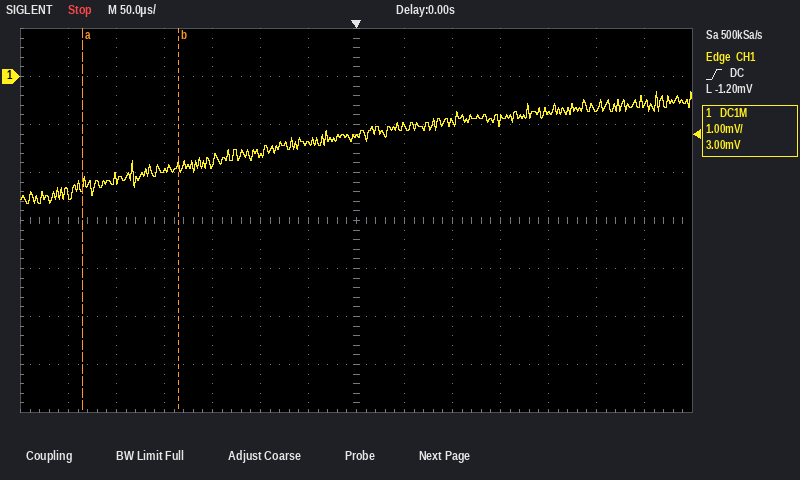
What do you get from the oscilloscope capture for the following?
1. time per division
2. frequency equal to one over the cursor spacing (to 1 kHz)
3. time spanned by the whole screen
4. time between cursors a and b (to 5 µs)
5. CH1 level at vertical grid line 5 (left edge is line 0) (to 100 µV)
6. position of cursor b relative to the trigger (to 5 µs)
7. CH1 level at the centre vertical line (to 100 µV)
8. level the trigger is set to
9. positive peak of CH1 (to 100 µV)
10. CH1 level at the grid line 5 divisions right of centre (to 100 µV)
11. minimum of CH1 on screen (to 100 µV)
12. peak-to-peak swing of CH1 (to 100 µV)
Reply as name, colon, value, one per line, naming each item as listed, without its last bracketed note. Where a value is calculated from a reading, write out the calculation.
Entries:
time per division: 50 µs
frequency equal to one over the cursor spacing: 1 / 100 µs ≈ 10 kHz
time spanned by the whole screen: 700 µs
time between cursors a and b: 100 µs
CH1 level at vertical grid line 5 (left edge is line 0): -1.6 mV
position of cursor b relative to the trigger: -185 µs
CH1 level at the centre vertical line: -1.2 mV
level the trigger is set to: -1.20 mV
positive peak of CH1: -300 µV
CH1 level at the grid line 5 divisions right of centre: -700 µV
minimum of CH1 on screen: -2.6 mV
peak-to-peak swing of CH1: -300 µV − (-2.6 mV) = 2.3 mV
